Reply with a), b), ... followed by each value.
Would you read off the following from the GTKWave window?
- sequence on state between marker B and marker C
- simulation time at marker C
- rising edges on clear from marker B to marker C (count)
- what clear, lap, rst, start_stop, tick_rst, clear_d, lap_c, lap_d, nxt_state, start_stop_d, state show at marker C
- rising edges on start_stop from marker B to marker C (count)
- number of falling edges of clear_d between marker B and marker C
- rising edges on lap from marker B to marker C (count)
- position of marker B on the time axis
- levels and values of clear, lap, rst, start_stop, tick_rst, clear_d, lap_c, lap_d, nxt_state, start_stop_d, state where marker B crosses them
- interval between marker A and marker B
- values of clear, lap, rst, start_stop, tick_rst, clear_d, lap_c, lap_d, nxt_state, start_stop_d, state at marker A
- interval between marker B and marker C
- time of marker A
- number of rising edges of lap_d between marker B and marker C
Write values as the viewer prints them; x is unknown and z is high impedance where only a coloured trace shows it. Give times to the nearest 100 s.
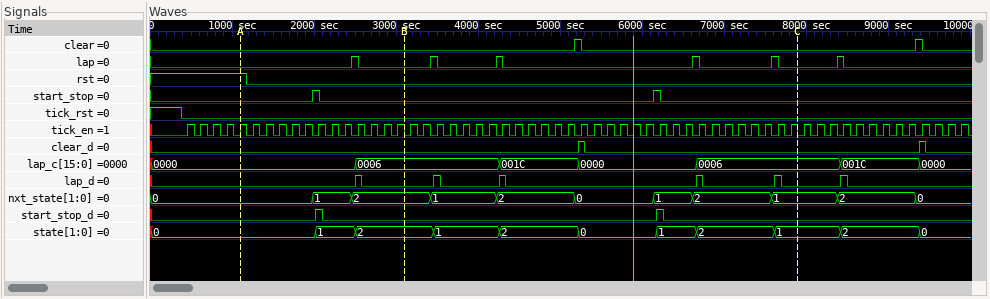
a) 2, 1, 2, 0, 1, 2, 1
b) 7900 s
c) 1
d) clear=0, lap=0, rst=0, start_stop=0, tick_rst=0, clear_d=0, lap_c=0006, lap_d=0, nxt_state=1, start_stop_d=0, state=1
e) 1
f) 1
g) 4
h) 3100 s
i) clear=0, lap=0, rst=0, start_stop=0, tick_rst=0, clear_d=0, lap_c=0006, lap_d=0, nxt_state=2, start_stop_d=0, state=2
j) 2000 s
k) clear=0, lap=0, rst=1, start_stop=0, tick_rst=0, clear_d=0, lap_c=0000, lap_d=0, nxt_state=0, start_stop_d=0, state=0
l) 4800 s
m) 1100 s
n) 4
